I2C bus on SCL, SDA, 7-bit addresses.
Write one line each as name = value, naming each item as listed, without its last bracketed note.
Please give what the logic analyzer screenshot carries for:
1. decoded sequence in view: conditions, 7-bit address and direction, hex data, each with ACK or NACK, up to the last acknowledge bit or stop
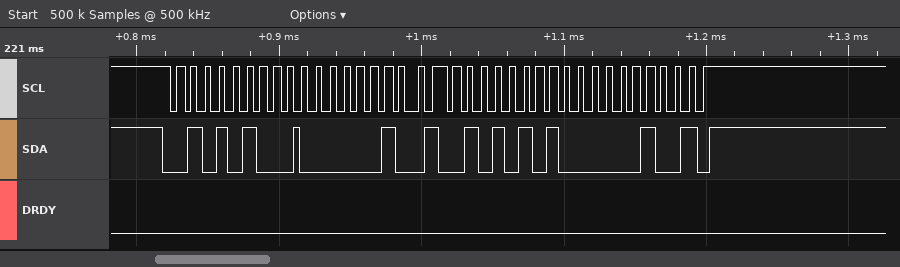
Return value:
decoded sequence in view: conditions, 7-bit address and direction, hex data, each with ACK or NACK, up to the last acknowledge bit or stop = start, address 2A write ACK, 02 ACK, repeated start, address 2A read ACK, 04 NACK, stop
